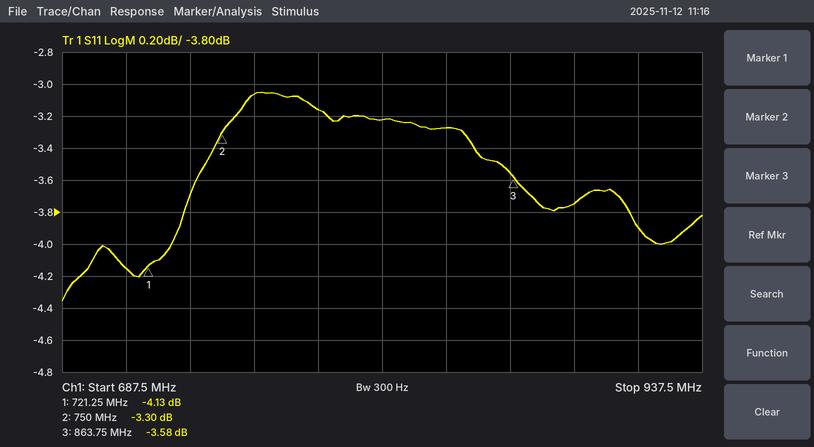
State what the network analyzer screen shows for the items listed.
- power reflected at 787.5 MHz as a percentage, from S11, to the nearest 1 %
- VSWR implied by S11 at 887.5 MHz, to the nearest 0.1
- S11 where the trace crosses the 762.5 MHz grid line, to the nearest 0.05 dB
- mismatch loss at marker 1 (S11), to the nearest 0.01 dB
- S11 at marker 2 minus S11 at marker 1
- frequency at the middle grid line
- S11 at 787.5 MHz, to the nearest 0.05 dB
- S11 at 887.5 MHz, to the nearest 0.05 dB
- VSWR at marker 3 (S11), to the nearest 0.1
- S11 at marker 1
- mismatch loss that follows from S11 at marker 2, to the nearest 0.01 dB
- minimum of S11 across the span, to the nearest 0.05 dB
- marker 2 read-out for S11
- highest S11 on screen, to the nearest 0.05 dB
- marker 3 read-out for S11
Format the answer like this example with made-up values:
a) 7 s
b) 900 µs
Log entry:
a) 48 %
b) 4.7
c) -3.05 dB
d) 2.12 dB
e) 0.83 dB
f) 812.5 MHz
g) -3.15 dB
h) -3.75 dB
i) 4.9
j) -4.13 dB
k) 2.74 dB
l) -4.35 dB
m) -3.30 dB
n) -3.05 dB
o) -3.58 dB
